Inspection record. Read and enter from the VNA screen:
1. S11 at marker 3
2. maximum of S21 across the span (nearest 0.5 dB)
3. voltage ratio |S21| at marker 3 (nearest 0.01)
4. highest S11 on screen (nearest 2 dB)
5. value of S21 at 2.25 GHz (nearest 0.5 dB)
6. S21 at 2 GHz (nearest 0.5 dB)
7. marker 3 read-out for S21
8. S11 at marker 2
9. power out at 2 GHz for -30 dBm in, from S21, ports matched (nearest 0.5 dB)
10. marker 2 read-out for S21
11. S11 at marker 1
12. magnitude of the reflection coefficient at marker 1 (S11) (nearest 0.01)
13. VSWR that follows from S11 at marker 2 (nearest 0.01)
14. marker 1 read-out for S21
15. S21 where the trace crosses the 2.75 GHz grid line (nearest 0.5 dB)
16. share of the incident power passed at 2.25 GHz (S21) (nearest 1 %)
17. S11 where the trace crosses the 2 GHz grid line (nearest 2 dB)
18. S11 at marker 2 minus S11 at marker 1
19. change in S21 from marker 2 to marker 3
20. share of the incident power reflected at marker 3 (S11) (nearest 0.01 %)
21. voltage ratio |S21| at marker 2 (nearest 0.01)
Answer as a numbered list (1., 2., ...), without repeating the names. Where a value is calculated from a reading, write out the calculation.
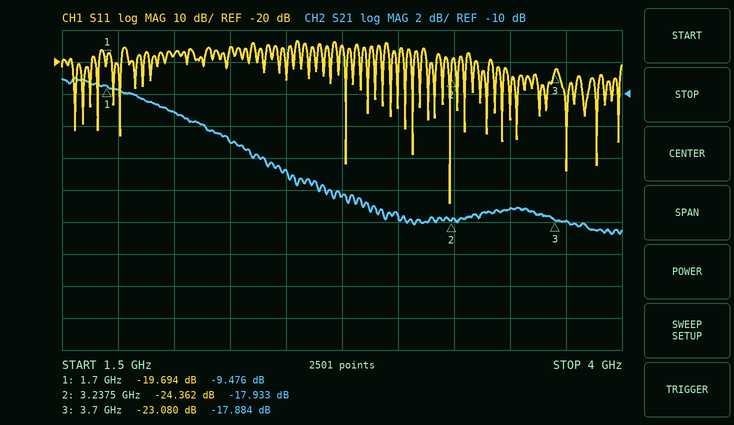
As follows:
1. -23.080 dB
2. -9.0 dB
3. 10^(-17.884/20) ≈ 0.13
4. -14 dB
5. -13.0 dB
6. -11.0 dB
7. -17.884 dB
8. -24.362 dB
9. -30 dBm + (-11.0 dB) = -41.0 dBm
10. -17.933 dB
11. -19.694 dB
12. 10^(-19.694/20) ≈ 0.10
13. (1 + 0.0605)/(1 − 0.0605) ≈ 1.13
14. -9.476 dB
15. -16.5 dB
16. 10^(-13/10) ≈ 5 %
17. -18 dB
18. -24.362 − (-19.694) = -4.668 dB
19. -17.884 − (-17.933) = 0.049 dB
20. 10^(-23.08/10) ≈ 0.49 %
21. 10^(-17.933/20) ≈ 0.13
